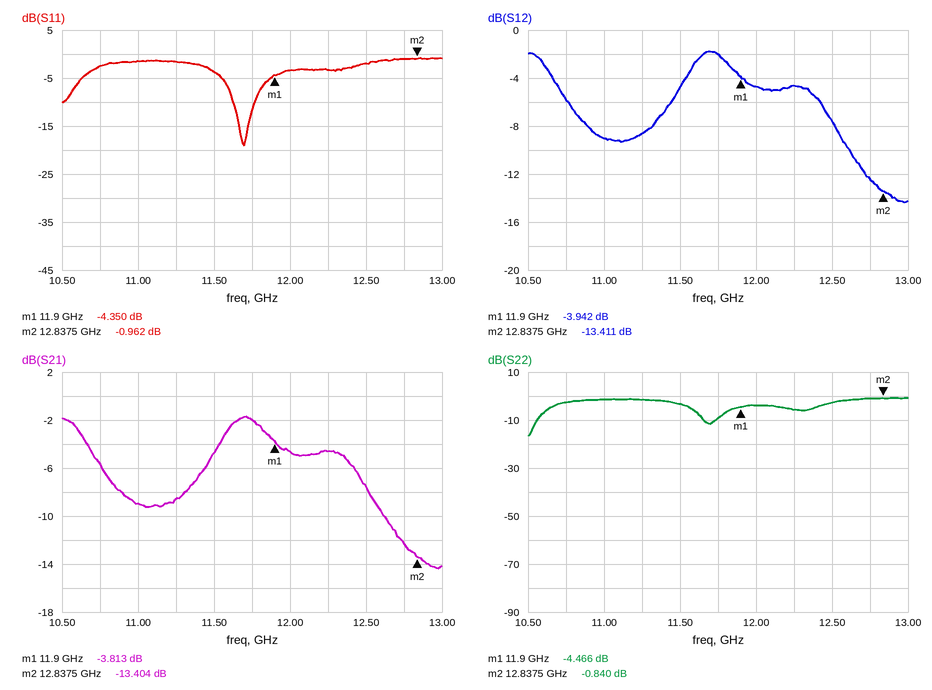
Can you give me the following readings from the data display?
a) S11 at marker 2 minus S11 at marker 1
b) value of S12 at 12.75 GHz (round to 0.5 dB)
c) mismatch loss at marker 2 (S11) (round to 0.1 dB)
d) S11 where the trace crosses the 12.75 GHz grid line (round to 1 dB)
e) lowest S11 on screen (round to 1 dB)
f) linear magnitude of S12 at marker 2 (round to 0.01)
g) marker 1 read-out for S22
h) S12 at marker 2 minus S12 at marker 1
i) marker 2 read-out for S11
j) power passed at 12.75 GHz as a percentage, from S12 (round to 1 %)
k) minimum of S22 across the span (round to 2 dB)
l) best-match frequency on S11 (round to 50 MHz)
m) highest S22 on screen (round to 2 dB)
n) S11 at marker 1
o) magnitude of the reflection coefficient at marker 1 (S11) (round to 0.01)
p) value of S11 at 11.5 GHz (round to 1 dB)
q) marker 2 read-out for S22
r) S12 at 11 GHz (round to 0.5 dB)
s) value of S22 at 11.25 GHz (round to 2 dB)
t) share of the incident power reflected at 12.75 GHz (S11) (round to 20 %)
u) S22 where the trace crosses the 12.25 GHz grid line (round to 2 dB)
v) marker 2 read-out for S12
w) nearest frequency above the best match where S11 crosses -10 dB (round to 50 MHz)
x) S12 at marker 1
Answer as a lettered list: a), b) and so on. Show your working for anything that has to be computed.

a) -0.962 − (-4.35) = 3.388 dB
b) -12.5 dB
c) −10 log10(1 − 10^(-0.962/10)) ≈ 7.0 dB
d) -1 dB
e) -19 dB
f) 10^(-13.411/20) ≈ 0.21
g) -4.466 dB
h) -13.411 − (-3.942) = -9.469 dB
i) -0.962 dB
j) 10^(-12.5/10) ≈ 6 %
k) -16 dB
l) 11.70 GHz
m) 0 dB
n) -4.350 dB
o) 10^(-4.35/20) ≈ 0.61
p) -4 dB
q) -0.840 dB
r) -9.0 dB
s) -2 dB
t) 10^(-1/10) ≈ 79.4 %, so 80 % to the nearest 20 %
u) -6 dB
v) -13.411 dB
w) 11.75 GHz
x) -3.942 dB
